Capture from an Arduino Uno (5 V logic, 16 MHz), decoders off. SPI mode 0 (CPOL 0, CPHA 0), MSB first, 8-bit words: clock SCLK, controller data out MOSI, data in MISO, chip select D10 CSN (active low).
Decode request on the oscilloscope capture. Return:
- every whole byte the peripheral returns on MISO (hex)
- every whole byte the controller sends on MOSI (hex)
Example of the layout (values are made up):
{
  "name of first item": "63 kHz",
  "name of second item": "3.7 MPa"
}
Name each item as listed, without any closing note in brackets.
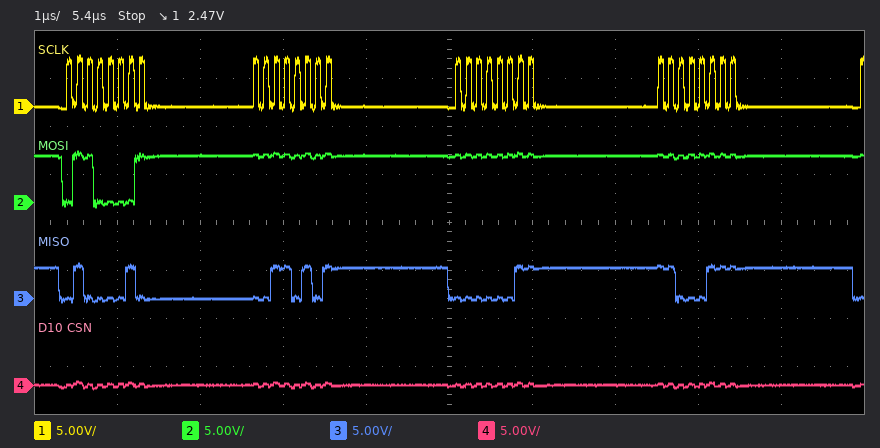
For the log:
{
  "every whole byte the peripheral returns on MISO": "42 35 03 C7",
  "every whole byte the controller sends on MOSI": "61 FF FF FF"
}
